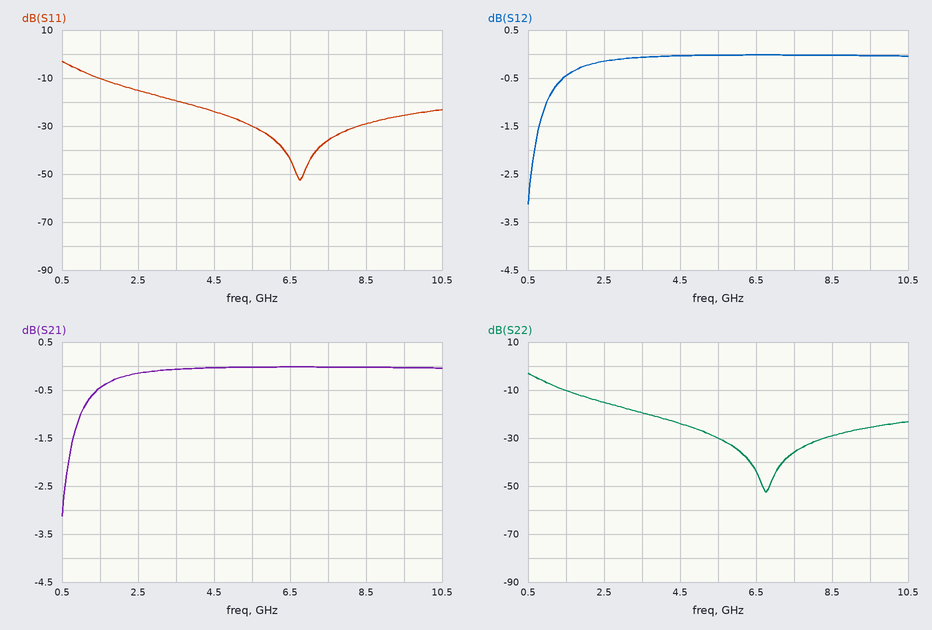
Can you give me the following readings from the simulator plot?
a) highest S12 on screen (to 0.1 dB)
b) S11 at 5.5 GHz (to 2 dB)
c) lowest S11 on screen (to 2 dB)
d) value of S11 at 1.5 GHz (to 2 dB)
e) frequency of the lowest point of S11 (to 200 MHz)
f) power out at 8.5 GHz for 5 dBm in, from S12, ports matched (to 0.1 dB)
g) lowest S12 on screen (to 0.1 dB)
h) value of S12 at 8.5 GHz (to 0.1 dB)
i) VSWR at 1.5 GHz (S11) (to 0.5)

0.0 dB
-30 dB
-52 dB
-10 dB
6.8 GHz
5.0 dBm
-3.1 dB
0.0 dB
2.0
